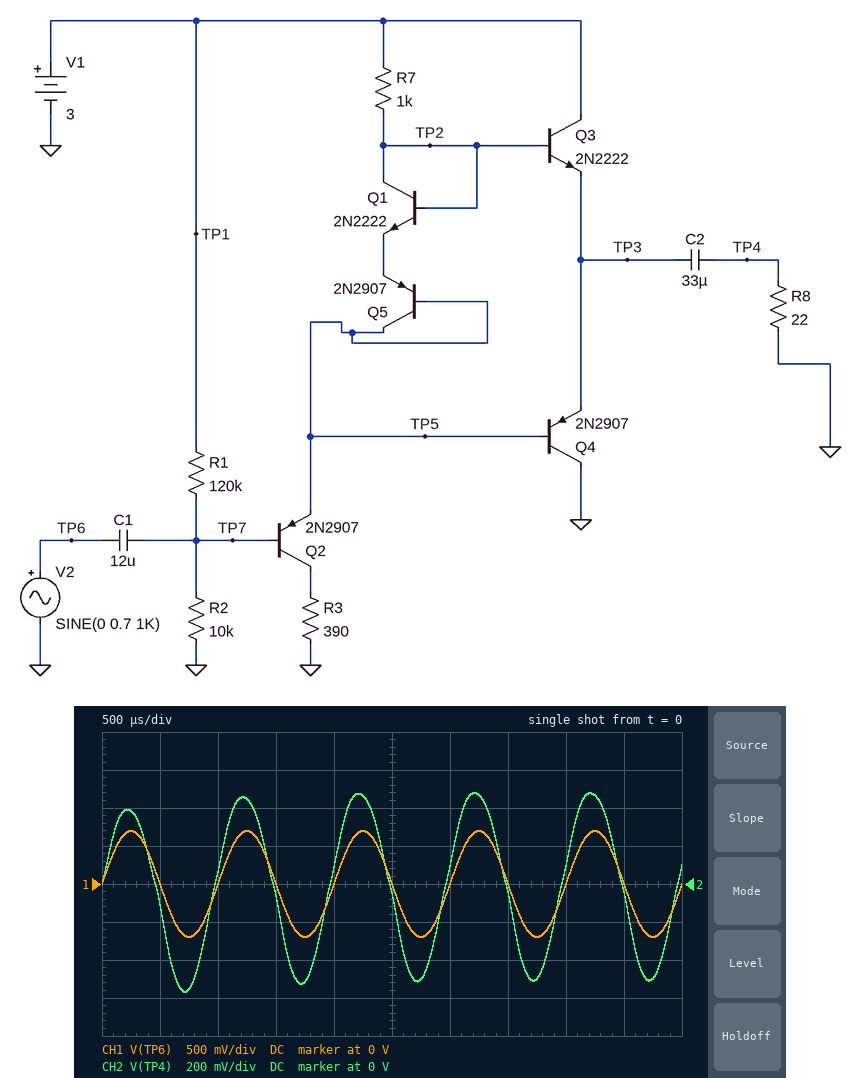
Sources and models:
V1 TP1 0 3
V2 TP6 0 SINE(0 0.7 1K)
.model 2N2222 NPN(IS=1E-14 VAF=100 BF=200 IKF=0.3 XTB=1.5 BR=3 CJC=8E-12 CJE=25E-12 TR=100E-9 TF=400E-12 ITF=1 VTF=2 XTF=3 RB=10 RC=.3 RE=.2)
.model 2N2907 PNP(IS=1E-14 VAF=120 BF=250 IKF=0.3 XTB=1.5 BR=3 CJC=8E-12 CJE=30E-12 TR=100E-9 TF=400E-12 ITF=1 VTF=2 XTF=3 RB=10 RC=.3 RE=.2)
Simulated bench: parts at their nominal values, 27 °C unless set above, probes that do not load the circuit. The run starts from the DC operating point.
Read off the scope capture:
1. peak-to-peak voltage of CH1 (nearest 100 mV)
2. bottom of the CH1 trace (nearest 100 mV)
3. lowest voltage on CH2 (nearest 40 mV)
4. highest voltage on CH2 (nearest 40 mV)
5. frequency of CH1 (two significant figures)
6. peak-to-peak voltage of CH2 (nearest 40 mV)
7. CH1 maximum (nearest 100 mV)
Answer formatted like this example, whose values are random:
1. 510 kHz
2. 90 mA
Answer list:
1. 1.4 V
2. -700 mV
3. -560 mV
4. 480 mV
5. 1.0 kHz
6. 1.04 V
7. 700 mV
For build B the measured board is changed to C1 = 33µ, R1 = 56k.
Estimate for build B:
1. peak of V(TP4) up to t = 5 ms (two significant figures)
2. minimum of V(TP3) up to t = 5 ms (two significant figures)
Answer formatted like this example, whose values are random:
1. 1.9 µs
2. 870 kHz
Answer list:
1. 420 mV
2. 1.2 V
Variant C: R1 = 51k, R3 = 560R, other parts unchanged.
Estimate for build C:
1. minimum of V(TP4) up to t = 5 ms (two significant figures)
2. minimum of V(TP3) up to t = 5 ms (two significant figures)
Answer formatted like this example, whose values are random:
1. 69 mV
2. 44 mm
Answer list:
1. -550 mV
2. 1.2 V
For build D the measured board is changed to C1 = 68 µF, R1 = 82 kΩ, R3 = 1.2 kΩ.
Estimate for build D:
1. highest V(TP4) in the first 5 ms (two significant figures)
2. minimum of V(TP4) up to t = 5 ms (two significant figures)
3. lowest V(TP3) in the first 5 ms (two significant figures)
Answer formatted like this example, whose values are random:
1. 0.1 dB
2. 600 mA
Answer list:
1. 450 mV
2. -560 mV
3. 1.1 V
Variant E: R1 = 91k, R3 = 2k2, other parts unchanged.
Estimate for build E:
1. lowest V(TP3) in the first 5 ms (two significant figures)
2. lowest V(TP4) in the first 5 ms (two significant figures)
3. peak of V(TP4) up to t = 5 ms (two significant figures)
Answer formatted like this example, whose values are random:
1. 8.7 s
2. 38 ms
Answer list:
1. 1.3 V
2. -530 mV
3. 370 mV
